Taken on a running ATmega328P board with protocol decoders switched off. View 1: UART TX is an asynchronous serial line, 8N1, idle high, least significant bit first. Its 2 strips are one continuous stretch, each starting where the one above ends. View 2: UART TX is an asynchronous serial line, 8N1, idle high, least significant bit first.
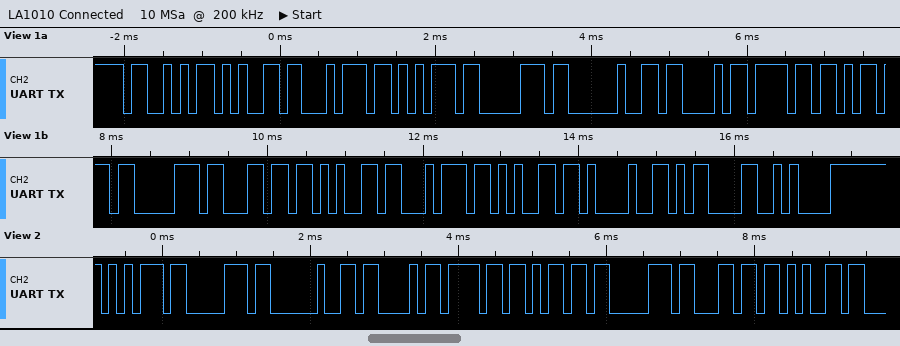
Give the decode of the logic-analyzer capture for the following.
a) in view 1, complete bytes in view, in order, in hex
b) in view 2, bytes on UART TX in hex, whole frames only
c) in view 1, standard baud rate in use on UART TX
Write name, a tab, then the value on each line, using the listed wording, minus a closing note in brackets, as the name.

in view 1, complete bytes in view, in order, in hex	0x53 0x65 0x74 0x75 0x70 0x20 0x43 0x6F 0x6D 0x70 0x6C 0x65 0x74 0x65 0x21 0x0D 0x0A
in view 2, bytes on UART TX in hex, whole frames only	75 70 20 43 6F 6D 70 6C 65
in view 1, standard baud rate in use on UART TX	9600 baud
